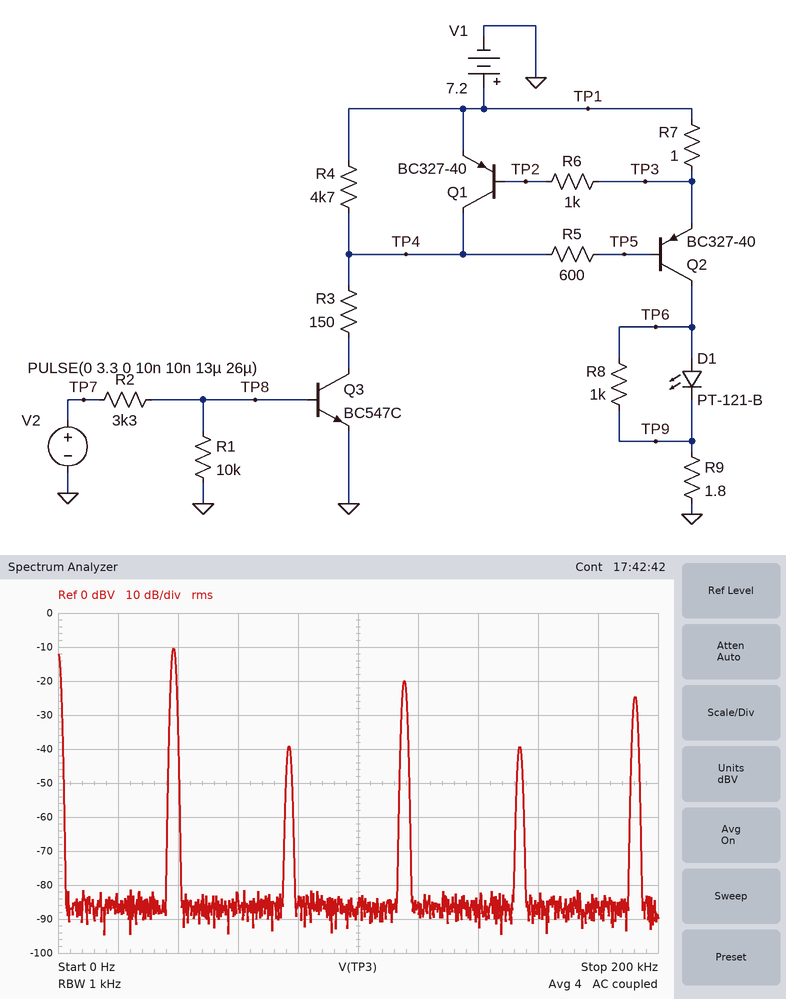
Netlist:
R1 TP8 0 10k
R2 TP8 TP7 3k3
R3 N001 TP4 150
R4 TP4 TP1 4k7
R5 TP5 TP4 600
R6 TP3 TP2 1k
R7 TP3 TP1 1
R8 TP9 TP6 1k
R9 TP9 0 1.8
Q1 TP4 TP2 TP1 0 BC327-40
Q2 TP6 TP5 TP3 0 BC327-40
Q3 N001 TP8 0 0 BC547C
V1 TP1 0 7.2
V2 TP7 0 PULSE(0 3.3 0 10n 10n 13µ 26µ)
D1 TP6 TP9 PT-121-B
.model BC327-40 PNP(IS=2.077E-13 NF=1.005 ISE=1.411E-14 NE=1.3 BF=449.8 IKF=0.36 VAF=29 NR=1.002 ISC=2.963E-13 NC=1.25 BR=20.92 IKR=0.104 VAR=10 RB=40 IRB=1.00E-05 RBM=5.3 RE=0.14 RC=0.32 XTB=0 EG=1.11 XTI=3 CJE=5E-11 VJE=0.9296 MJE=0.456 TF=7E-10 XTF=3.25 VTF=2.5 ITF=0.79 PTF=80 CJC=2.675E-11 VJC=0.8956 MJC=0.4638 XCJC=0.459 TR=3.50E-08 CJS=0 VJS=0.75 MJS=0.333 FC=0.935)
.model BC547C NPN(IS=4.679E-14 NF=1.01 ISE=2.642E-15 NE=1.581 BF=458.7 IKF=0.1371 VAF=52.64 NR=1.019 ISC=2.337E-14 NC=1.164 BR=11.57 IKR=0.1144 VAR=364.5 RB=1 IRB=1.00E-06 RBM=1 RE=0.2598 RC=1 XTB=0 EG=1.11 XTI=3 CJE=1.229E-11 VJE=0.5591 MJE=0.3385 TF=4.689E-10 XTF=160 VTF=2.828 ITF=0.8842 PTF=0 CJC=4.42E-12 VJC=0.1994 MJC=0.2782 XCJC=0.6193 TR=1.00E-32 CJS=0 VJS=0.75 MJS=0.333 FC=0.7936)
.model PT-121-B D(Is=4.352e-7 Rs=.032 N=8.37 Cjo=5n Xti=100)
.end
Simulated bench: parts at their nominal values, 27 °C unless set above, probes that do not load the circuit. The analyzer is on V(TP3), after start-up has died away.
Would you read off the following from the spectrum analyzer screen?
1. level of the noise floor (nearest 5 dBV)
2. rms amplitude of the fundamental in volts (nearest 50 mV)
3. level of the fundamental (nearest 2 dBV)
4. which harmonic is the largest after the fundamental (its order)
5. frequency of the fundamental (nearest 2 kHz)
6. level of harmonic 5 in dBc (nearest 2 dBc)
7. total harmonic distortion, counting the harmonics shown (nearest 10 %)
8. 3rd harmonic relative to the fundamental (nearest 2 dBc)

-85 dBV
300 mV
-10 dBV
3
38 kHz
-14 dBc
40 %
-10 dBc
